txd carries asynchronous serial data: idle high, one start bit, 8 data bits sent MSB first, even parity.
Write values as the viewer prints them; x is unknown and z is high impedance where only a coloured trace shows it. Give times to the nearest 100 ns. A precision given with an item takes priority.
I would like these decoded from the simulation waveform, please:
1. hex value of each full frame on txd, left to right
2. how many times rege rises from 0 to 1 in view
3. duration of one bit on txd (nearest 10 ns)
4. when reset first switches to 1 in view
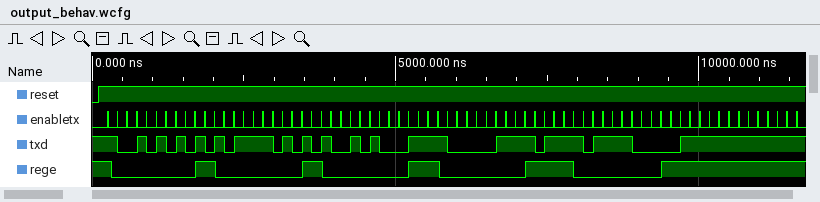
55, F5, 51, 0F, F0
5
160 ns
100 ns
